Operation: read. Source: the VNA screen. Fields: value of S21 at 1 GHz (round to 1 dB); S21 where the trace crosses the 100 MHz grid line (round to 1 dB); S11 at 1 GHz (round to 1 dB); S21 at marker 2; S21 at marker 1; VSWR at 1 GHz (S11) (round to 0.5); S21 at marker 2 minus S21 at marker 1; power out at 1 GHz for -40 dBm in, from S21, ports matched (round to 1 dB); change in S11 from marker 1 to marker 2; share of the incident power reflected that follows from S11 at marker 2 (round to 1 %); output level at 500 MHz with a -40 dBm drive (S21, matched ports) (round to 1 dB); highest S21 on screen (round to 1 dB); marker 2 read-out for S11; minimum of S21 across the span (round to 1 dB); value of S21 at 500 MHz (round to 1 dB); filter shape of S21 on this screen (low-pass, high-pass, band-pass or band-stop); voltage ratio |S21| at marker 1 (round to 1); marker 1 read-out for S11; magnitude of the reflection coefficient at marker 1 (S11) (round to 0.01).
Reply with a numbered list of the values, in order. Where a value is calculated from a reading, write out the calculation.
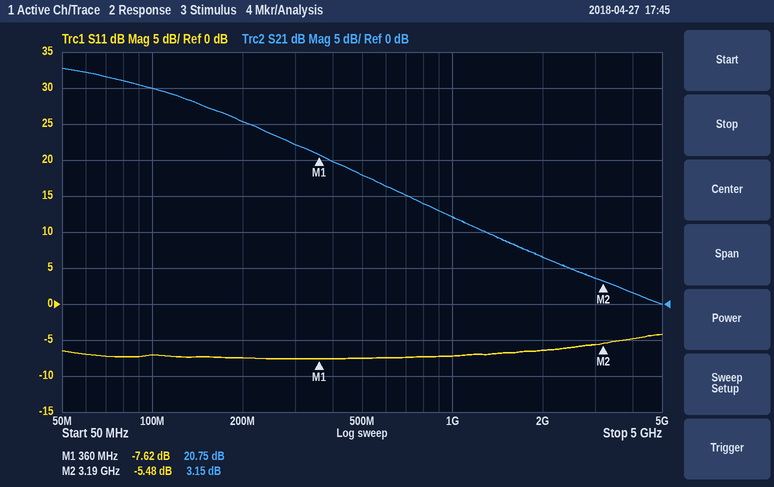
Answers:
1. 12 dB
2. 30 dB
3. -7 dB
4. 3.15 dB
5. 20.75 dB
6. |Γ| = 10^(-7/20) = 0.4467; VSWR = (1 + 0.4467)/(1 − 0.4467) ≈ 2.61, so 2.5 to the nearest 0.5
7. 3.15 − (20.75) = -17.60 dB
8. -40 dBm + (12 dB) = -28 dBm
9. -5.48 − (-7.62) = 2.14 dB
10. 10^(-5.48/10) ≈ 28 %
11. -40 dBm + (18 dB) = -22 dBm
12. 33 dB
13. -5.48 dB
14. 0 dB
15. 18 dB
16. low-pass
17. 10^(20.75/20) ≈ 11
18. -7.62 dB
19. 10^(-7.62/20) ≈ 0.42
